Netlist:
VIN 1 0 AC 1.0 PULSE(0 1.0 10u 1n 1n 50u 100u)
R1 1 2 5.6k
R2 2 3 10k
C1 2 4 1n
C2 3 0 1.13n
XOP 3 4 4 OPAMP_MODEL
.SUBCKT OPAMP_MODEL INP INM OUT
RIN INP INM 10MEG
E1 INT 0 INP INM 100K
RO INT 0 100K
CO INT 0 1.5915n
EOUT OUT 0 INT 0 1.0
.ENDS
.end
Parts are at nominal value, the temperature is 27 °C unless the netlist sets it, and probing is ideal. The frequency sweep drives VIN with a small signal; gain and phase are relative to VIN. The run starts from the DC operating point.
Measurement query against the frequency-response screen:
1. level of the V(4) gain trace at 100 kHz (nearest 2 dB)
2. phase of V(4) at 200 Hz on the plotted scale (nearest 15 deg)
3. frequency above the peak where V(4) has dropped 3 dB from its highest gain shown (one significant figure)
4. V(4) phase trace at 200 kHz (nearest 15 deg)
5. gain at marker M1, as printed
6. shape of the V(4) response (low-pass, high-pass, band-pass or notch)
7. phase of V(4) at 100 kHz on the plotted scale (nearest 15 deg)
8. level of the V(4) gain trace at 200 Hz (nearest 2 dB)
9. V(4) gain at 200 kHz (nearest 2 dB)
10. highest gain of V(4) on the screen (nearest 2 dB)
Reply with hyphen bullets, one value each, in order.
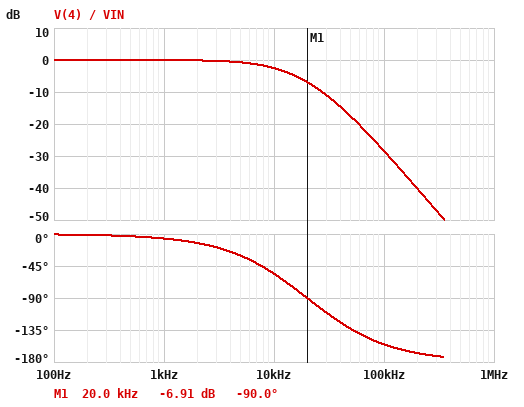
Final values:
- -28 dB
- 0 deg
- 10 kHz
- -165 deg
- -6.91 dB
- low-pass
- -150 deg
- 0 dB
- -40 dB
- 0 dB
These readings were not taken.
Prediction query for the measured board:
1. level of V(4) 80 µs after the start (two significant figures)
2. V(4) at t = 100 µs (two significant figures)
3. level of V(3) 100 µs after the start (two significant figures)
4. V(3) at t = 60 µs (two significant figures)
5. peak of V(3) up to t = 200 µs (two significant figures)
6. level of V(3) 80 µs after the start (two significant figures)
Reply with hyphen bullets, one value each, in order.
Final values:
- 320 mV
- 68 mV
- 68 mV
- 970 mV
- 970 mV
- 320 mV
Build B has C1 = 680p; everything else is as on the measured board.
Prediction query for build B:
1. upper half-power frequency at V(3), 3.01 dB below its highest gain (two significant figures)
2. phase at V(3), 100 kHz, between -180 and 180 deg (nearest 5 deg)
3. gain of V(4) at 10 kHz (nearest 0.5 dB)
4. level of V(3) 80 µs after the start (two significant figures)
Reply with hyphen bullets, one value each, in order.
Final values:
- 10 kHz
- -145 deg
- -3.0 dB
- 310 mV
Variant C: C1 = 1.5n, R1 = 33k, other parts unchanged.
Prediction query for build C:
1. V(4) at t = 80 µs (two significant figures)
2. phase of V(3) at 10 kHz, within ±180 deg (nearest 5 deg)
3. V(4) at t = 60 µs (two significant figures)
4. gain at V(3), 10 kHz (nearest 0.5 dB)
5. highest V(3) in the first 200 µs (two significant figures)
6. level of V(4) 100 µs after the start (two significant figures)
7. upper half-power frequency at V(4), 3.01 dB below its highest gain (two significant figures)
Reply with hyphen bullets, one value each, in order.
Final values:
- 580 mV
- -110 deg
- 610 mV
- -10.5 dB
- 700 mV
- 390 mV
- 4.2 kHz
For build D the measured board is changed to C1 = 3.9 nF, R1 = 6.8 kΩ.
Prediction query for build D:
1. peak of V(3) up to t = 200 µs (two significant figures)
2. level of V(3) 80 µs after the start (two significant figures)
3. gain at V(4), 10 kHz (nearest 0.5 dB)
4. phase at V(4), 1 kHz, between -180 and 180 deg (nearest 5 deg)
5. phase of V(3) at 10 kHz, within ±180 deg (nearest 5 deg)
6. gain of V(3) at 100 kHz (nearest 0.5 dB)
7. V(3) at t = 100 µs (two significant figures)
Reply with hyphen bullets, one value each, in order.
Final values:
- 1.1 V
- 710 mV
- -1.5 dB
- -5 deg
- -100 deg
- -41.5 dB
- 130 mV
